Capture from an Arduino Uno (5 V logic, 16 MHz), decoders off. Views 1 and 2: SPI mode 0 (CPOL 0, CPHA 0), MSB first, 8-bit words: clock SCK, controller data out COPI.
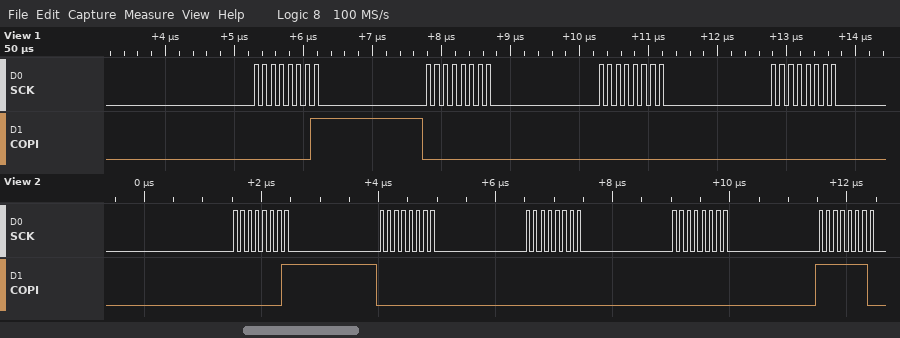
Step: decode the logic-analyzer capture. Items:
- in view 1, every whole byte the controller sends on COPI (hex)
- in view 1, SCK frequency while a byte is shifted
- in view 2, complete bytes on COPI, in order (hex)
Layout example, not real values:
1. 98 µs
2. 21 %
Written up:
1. 0x01 0x00 0x00 0x00
2. 8 MHz
3. 0x01 0x00 0x00 0x00 0xFE
